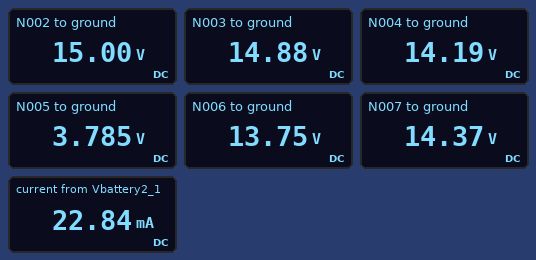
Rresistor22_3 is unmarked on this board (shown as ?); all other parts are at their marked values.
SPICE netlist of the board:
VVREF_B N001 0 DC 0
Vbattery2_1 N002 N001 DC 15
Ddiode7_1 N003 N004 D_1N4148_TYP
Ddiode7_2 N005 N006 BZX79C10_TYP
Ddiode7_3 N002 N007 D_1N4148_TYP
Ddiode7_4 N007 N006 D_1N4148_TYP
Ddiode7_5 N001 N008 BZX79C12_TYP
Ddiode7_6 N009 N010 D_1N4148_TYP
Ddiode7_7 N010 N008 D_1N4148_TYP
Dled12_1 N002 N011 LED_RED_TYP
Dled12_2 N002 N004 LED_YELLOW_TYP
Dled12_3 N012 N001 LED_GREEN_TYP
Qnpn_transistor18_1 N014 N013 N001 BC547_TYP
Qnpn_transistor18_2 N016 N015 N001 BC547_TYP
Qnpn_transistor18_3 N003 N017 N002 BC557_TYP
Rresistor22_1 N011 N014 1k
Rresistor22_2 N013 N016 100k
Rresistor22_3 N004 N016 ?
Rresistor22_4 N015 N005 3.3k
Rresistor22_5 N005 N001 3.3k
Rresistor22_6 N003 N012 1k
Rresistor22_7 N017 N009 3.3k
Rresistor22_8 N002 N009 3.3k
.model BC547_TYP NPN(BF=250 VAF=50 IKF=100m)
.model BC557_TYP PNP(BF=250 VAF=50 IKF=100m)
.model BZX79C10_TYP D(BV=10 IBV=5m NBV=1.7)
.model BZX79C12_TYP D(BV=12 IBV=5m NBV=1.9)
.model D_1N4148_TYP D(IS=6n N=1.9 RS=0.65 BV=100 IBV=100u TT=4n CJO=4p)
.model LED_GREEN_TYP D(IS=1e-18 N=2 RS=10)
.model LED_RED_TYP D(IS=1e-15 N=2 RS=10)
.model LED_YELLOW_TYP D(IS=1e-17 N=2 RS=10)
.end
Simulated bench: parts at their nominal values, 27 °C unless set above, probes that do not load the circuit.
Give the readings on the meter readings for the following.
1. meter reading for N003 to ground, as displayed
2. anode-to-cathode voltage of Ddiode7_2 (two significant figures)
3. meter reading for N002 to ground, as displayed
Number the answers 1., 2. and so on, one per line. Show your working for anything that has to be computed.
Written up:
1. 14.88 V
2. 3.785 V - 13.75 V = -10 V
3. 15.00 V
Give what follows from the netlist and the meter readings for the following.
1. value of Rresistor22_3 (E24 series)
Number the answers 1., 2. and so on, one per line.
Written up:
1. 2 kΩ
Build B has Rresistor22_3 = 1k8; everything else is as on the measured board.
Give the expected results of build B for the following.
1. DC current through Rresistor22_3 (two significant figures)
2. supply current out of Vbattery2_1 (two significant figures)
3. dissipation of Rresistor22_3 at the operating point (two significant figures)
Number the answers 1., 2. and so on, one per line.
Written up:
1. 7.8 mA
2. 24 mA
3. 110 mW
